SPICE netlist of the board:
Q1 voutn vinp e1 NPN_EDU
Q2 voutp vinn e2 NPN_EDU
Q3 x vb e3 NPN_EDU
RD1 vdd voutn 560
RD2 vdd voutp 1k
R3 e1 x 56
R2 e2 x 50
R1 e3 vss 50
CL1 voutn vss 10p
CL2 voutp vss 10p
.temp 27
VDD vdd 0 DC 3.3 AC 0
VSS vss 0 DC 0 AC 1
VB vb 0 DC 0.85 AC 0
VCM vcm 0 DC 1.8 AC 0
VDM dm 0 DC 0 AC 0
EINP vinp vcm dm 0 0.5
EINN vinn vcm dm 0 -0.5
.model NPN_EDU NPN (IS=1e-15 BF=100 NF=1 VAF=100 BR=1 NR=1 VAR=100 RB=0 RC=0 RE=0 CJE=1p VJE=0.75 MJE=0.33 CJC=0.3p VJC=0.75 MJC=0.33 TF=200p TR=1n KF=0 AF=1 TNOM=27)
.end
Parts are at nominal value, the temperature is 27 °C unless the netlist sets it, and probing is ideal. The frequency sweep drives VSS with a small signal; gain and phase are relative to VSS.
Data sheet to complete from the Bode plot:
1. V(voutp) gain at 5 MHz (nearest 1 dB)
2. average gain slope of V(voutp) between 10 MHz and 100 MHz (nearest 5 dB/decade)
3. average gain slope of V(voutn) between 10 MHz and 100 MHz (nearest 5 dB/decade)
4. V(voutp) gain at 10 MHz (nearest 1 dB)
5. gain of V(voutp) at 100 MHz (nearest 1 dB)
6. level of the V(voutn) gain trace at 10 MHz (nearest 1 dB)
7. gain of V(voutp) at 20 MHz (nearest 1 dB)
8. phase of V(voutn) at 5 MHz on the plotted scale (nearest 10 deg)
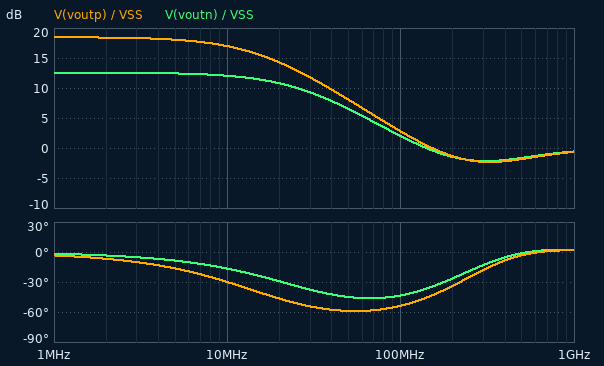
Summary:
18 dB
-15 dB/decade
-10 dB/decade
17 dB
3 dB
12 dB
14 dB
-10 deg
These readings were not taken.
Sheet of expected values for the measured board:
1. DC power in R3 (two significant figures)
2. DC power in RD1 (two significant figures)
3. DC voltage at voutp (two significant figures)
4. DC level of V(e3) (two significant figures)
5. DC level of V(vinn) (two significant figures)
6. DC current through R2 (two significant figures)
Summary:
66 µW
650 µW
2.1 V
110 mV
1.8 V
1.2 mA
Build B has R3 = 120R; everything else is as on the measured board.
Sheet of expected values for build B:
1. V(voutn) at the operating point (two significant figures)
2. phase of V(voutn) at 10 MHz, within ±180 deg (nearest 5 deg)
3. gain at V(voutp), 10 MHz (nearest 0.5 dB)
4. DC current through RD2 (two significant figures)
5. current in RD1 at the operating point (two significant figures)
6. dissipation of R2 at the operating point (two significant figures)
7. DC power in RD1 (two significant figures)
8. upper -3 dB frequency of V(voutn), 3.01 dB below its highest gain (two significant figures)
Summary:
2.9 V
-15 deg
19.5 dB
1.5 mA
760 µA
110 µW
320 µW
30 MHz
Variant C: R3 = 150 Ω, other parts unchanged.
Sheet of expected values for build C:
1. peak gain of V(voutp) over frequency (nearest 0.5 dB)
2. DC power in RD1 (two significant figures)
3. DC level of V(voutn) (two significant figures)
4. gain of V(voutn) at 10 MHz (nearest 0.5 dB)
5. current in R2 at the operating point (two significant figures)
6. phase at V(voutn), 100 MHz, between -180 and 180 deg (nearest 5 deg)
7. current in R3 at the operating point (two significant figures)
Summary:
21.5 dB
250 µW
2.9 V
7.0 dB
1.6 mA
-20 deg
680 µA
